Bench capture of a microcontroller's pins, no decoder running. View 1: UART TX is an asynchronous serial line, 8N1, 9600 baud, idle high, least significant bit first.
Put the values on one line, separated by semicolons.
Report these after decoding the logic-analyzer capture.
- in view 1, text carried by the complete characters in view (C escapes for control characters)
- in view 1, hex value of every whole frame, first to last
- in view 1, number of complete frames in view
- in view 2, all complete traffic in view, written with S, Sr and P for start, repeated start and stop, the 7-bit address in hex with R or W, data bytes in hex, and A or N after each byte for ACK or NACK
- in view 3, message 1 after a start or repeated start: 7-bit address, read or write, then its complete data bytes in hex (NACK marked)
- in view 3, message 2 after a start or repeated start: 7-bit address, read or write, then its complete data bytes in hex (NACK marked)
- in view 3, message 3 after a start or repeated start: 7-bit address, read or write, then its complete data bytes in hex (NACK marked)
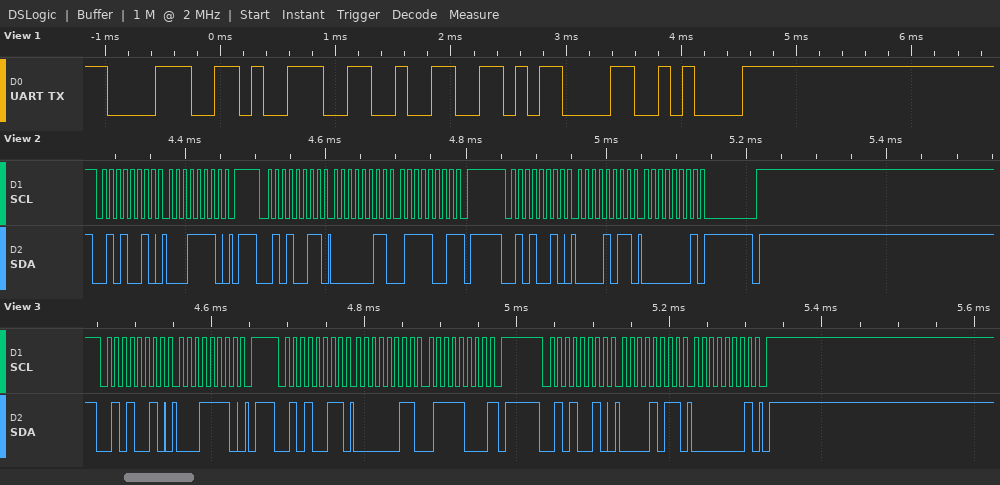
"892\r\n"; 38 39 32 0D 0A; 5; S 29W A 1E A P S 29R A 03 A 79 N P S 29W A 0B A 01 A P; 0x29 write: 1E; 0x29 read: 03 78 NACK; 0x29 write: 0B 01
